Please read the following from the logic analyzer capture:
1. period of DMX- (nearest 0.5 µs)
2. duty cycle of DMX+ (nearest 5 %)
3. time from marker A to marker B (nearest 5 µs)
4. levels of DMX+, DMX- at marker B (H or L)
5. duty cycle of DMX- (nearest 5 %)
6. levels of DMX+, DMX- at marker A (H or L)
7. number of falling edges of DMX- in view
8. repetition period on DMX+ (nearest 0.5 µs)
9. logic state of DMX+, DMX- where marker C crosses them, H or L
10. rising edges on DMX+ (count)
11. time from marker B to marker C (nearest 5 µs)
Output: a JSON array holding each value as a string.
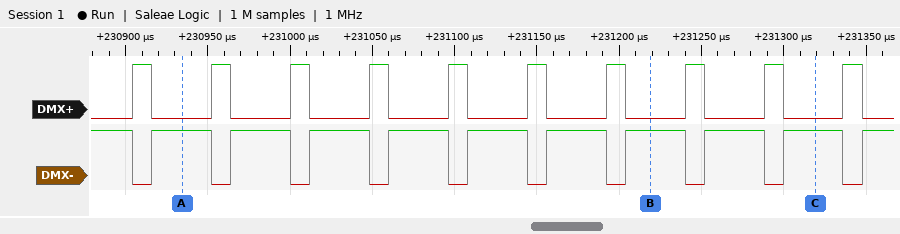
["48 µs", "25 %", "285 µs", "DMX+=L, DMX-=H", "75 %", "DMX+=L, DMX-=H", "10", "48 µs", "DMX+=L, DMX-=H", "10", "100 µs"]
